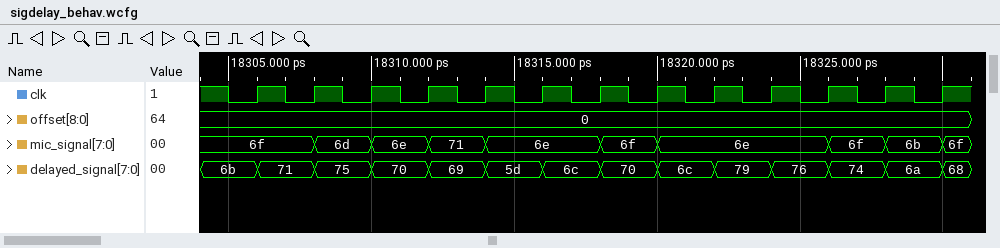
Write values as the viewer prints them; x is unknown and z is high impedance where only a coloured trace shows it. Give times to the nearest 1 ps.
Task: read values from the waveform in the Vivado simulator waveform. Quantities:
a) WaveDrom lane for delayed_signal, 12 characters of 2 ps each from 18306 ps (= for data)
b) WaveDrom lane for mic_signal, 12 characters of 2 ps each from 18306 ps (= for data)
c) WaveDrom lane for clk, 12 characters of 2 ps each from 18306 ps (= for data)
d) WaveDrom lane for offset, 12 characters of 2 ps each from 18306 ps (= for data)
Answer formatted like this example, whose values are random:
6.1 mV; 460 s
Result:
{name: 'delayed_signal', wave: '============', data: '71 75 70 69 5d 6c 70 6c 79 76 74 6a'}; {name: 'mic_signal', wave: '=====.==..==', data: '6f 6d 6e 71 6e 6f 6e 6f 6b'}; {name: 'clk', wave: 'p...........'}; {name: 'offset', wave: '=...........', data: '0'}
